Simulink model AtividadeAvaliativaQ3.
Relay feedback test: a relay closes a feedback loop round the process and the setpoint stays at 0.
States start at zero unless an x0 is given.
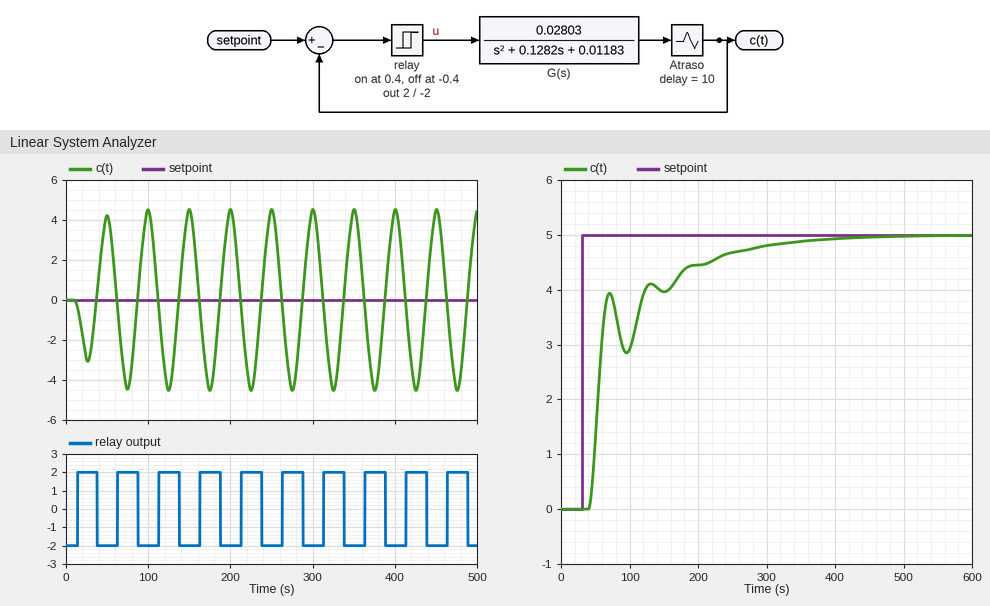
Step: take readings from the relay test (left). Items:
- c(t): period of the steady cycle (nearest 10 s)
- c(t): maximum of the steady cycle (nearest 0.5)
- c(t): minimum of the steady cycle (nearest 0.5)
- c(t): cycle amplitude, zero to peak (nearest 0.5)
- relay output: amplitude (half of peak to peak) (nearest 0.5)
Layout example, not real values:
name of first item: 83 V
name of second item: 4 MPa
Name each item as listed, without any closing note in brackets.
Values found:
c(t): period of the steady cycle: 50 s
c(t): maximum of the steady cycle: 4.5
c(t): minimum of the steady cycle: -4.5
c(t): cycle amplitude, zero to peak: 4.5
relay output: amplitude (half of peak to peak): 2.0
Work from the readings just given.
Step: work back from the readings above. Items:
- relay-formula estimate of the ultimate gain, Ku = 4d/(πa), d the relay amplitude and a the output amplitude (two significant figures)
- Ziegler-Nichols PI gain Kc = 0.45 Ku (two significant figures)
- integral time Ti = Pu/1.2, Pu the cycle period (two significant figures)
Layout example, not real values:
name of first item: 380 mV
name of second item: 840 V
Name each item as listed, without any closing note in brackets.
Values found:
relay-formula estimate of the ultimate gain, Ku = 4d/(πa), d the relay amplitude and a the output amplitude: 0.57
Ziegler-Nichols PI gain Kc = 0.45 Ku: 0.26
integral time Ti = Pu/1.2, Pu the cycle period: 42 s
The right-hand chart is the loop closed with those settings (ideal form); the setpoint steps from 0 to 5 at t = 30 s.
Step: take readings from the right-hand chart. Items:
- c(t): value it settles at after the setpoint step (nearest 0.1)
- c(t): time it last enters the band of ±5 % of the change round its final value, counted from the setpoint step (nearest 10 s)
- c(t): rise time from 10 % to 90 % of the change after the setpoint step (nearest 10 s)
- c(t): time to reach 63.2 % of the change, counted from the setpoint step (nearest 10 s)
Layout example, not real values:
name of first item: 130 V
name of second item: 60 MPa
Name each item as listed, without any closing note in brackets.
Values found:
c(t): value it settles at after the setpoint step: 5.0
c(t): time it last enters the band of ±5 % of the change round its final value, counted from the setpoint step: 250 s
c(t): rise time from 10 % to 90 % of the change after the setpoint step: 170 s
c(t): time to reach 63.2 % of the change, counted from the setpoint step: 30 s
